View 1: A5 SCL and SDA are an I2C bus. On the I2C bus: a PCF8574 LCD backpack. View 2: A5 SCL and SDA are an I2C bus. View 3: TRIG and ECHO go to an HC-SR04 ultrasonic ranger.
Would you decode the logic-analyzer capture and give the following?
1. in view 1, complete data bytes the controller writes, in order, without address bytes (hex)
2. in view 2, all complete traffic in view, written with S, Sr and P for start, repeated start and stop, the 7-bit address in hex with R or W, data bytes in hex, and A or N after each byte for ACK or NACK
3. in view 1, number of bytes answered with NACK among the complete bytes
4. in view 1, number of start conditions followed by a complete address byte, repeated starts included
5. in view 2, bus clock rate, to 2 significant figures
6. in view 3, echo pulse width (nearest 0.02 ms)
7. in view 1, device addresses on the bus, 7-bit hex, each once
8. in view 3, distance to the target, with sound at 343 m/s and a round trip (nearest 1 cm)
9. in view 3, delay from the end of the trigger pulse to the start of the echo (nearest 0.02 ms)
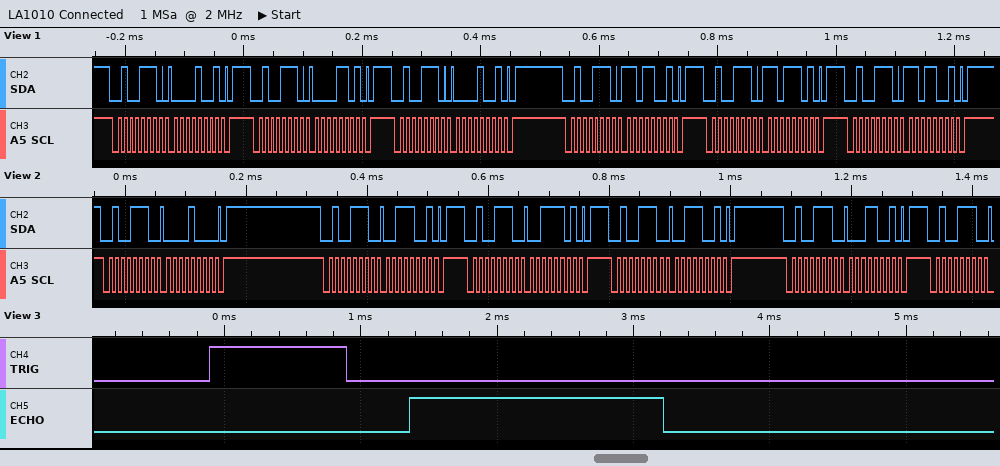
09 0D 09 D9 DD D9
S 27W A 08 A P S 27W A 39 A P S 27W A 3D A P S 27W A 39 A P S 27W A 19 A P S 27W A
0
6
100 kHz
1.86 ms
0x27
32 cm
0.46 ms
